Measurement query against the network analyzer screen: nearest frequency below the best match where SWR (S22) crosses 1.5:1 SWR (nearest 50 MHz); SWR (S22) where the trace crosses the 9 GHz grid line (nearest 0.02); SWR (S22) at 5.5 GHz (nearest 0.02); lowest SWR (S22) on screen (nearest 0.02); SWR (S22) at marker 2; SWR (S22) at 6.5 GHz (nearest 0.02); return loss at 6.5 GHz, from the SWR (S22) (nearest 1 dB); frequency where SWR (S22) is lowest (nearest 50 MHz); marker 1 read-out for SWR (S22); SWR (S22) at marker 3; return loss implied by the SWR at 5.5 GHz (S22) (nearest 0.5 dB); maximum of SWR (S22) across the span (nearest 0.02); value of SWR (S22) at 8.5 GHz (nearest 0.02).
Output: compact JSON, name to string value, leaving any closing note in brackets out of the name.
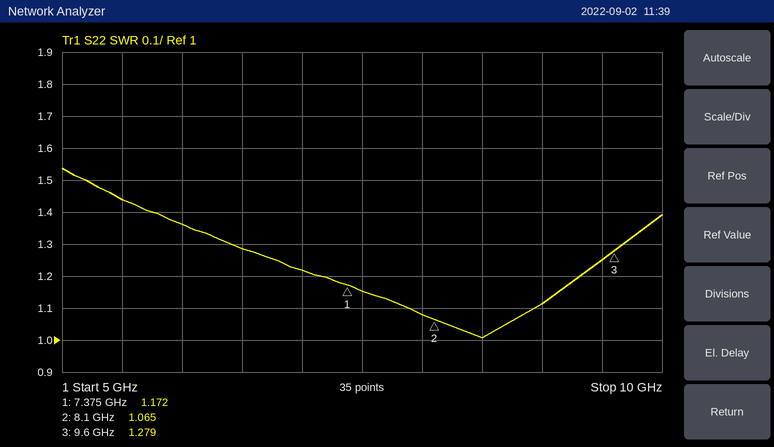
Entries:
{"nearest frequency below the best match where SWR (S22) crosses 1.5:1 SWR": "5.20 GHz", "SWR (S22) where the trace crosses the 9 GHz grid line": "1.12", "SWR (S22) at 5.5 GHz": "1.44", "lowest SWR (S22) on screen": "1.00", "SWR (S22) at marker 2": "1.065", "SWR (S22) at 6.5 GHz": "1.28", "return loss at 6.5 GHz, from the SWR (S22)": "18 dB", "frequency where SWR (S22) is lowest": "8.50 GHz", "marker 1 read-out for SWR": "1.172", "SWR (S22) at marker 3": "1.279", "return loss implied by the SWR at 5.5 GHz (S22)": "15.0 dB", "maximum of SWR (S22) across the span": "1.54", "value of SWR (S22) at 8.5 GHz": "1.00"}
